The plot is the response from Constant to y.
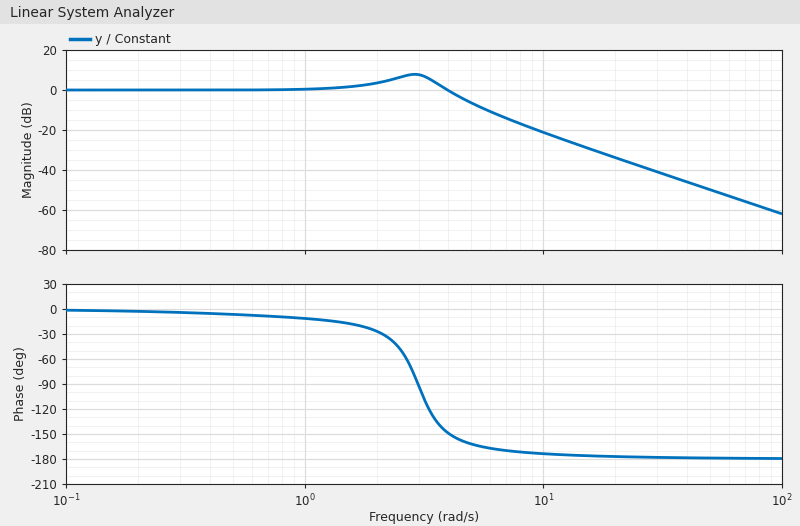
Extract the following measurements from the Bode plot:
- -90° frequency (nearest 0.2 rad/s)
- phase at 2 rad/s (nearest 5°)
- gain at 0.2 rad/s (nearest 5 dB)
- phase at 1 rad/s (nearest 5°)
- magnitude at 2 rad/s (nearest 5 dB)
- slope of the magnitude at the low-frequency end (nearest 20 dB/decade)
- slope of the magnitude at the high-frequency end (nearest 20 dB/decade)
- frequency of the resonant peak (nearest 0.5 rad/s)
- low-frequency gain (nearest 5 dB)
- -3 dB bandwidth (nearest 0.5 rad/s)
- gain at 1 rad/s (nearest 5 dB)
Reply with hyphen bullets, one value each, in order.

- 3.0 rad/s
- -25°
- 0 dB
- -10°
- 5 dB
- 0 dB/decade
- -40 dB/decade
- 3.0 rad/s
- 0 dB
- 4.5 rad/s
- 0 dB
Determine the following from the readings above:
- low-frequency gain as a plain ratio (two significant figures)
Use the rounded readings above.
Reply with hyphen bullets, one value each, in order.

- 1.0
